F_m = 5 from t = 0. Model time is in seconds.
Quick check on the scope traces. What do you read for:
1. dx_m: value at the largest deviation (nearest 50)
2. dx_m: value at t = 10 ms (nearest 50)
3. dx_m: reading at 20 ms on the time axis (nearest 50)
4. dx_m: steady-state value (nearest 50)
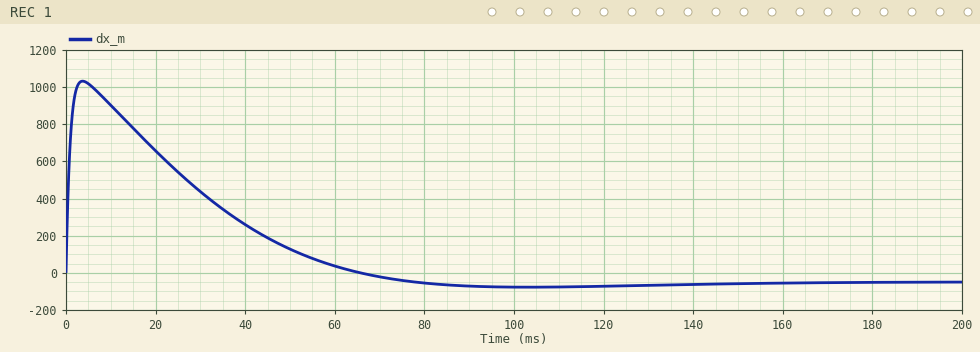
1050
900
650
-50
